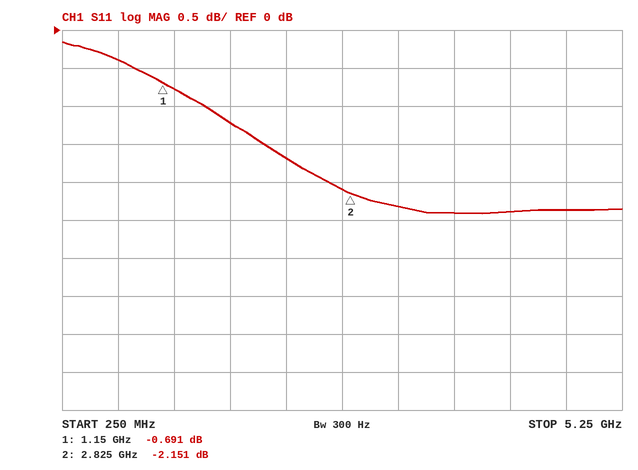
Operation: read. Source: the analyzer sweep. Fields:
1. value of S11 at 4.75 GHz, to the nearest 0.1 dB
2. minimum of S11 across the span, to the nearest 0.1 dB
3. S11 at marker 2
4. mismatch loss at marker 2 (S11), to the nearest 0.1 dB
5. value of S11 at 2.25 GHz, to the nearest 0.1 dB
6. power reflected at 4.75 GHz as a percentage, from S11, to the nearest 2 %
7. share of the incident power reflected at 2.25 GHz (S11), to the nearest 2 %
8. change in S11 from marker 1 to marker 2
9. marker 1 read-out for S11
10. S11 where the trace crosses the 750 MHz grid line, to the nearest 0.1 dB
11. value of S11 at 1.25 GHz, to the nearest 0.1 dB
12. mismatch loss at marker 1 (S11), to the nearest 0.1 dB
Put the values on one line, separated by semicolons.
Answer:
-2.4 dB; -2.4 dB; -2.151 dB; 4.1 dB; -1.7 dB; 58 %; 68 %; -1.460 dB; -0.691 dB; -0.4 dB; -0.8 dB; 8.3 dB
